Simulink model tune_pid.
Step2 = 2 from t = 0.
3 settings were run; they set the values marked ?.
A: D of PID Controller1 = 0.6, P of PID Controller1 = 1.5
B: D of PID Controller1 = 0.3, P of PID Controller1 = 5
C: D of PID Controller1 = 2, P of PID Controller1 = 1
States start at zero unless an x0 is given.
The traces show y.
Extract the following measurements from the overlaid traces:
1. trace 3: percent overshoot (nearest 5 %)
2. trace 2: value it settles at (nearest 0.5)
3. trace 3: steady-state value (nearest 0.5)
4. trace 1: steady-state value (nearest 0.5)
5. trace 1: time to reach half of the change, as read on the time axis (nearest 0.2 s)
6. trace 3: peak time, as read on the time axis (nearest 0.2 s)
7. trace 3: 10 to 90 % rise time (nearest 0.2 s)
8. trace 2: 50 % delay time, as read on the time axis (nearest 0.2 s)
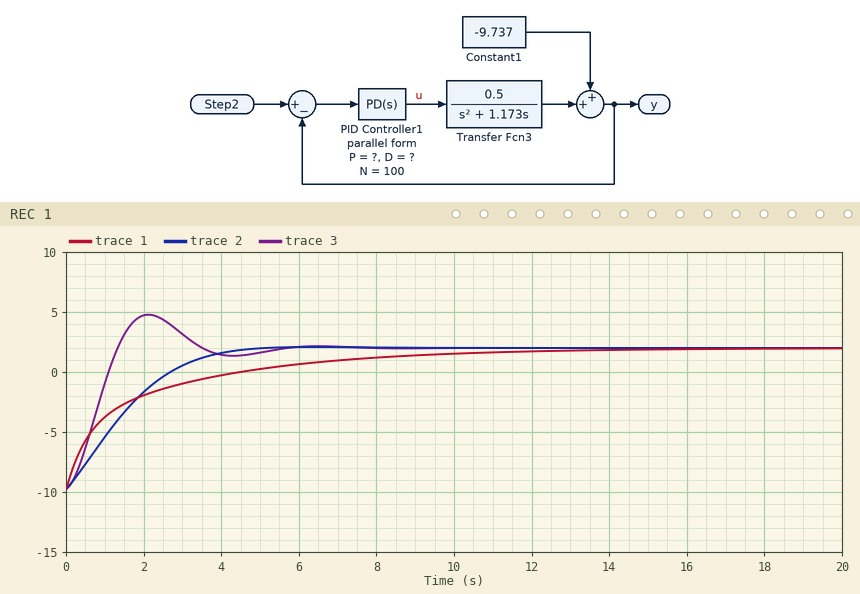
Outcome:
25 %
2.0
2.0
2.0
1.0 s
2.2 s
1.0 s
1.4 s
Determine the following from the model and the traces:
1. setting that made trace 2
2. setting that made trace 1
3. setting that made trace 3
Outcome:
A
C
B
